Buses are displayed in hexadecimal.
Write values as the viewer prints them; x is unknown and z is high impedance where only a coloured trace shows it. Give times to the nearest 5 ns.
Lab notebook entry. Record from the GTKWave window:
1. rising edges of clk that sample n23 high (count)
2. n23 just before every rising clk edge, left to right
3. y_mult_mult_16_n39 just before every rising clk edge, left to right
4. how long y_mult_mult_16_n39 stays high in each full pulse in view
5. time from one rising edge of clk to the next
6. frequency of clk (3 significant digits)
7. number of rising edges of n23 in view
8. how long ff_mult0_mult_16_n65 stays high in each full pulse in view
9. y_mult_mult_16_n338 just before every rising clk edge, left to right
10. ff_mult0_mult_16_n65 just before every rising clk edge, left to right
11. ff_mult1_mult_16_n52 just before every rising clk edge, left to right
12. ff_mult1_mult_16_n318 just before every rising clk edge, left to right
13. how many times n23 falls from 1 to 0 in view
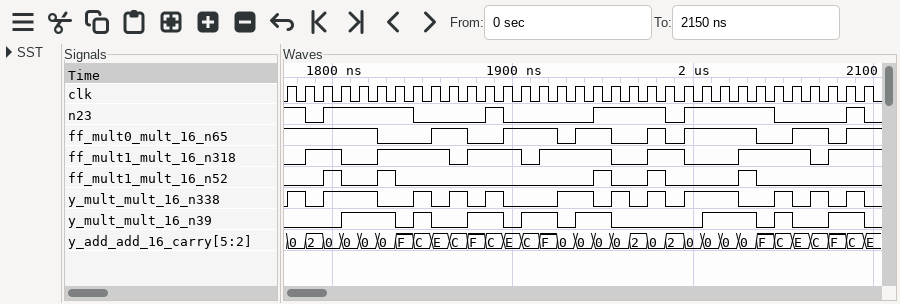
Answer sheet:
18
1 1 0 1 1 1 1 1 0 0 0 0 1 0 0 0 0 0 1 1 1 1 0 1 1 1 1 1 0 0 0 0 1
0 0 0 0 1 1 1 0 1 0 0 1 1 0 1 1 0 1 1 0 0 0 0 0 1 1 1 0 1 0 0 1 1
30 ns, 10 ns, 20 ns, 20 ns, 20 ns, 30 ns, 10 ns, 20 ns
10 ns
100 MHz
5
20 ns, 30 ns, 20 ns, 10 ns, 40 ns, 20 ns
0 1 0 1 1 1 0 0 1 0 1 0 1 0 0 0 1 1 0 1 0 1 0 1 1 1 0 0 1 0 1 0 1
1 1 1 1 1 1 0 0 0 1 1 0 0 1 1 1 0 1 1 0 0 1 0 1 1 1 1 0 0 1 1 0 1
0 0 0 1 0 0 1 0 0 0 0 0 0 0 0 0 0 0 1 0 0 1 0 0 0 0 1 0 0 0 0 0 0
0 0 1 1 0 0 1 1 1 1 0 1 1 1 0 1 1 1 1 0 0 1 1 0 0 0 1 1 1 1 0 1 1
6
